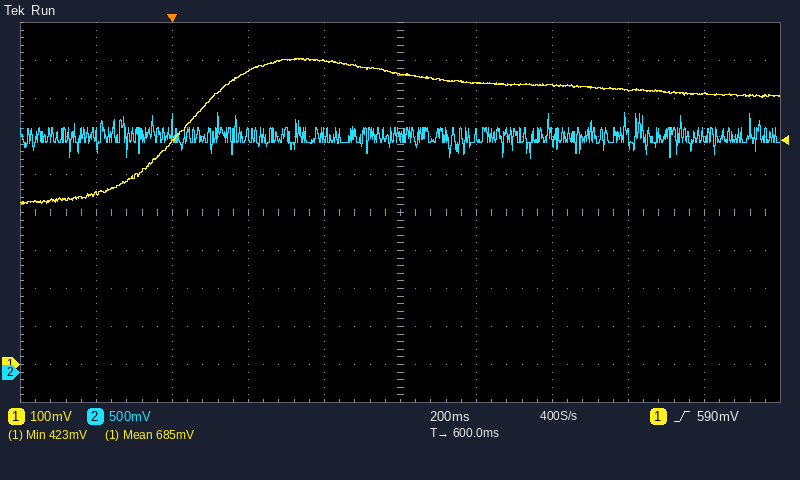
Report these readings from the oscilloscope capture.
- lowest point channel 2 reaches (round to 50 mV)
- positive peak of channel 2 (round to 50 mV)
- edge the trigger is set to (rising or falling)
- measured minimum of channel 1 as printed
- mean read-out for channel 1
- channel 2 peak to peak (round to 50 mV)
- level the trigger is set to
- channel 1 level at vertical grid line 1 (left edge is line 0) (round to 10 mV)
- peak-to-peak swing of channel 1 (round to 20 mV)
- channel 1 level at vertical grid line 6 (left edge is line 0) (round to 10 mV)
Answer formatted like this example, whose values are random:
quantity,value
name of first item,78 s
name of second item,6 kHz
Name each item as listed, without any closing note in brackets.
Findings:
quantity,value
lowest point channel 2 reaches,2.80 V
positive peak of channel 2,3.40 V
edge the trigger is set to,rising
measured minimum of channel 1 as printed,423 mV
mean read-out for channel 1,685 mV
channel 2 peak to peak,600 mV
level the trigger is set to,590 mV
channel 1 level at vertical grid line 1 (left edge is line 0),450 mV
peak-to-peak swing of channel 1,380 mV
channel 1 level at vertical grid line 6 (left edge is line 0),740 mV
